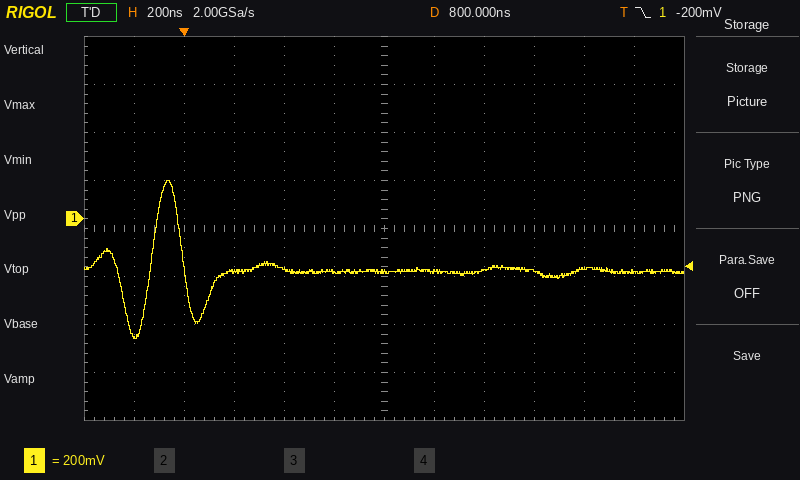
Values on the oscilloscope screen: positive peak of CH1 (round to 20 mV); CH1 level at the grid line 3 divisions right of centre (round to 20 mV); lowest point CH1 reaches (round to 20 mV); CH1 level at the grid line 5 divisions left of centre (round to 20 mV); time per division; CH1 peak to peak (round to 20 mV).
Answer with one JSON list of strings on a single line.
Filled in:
["160 mV", "-220 mV", "-500 mV", "-480 mV", "200 ns", "660 mV"]
